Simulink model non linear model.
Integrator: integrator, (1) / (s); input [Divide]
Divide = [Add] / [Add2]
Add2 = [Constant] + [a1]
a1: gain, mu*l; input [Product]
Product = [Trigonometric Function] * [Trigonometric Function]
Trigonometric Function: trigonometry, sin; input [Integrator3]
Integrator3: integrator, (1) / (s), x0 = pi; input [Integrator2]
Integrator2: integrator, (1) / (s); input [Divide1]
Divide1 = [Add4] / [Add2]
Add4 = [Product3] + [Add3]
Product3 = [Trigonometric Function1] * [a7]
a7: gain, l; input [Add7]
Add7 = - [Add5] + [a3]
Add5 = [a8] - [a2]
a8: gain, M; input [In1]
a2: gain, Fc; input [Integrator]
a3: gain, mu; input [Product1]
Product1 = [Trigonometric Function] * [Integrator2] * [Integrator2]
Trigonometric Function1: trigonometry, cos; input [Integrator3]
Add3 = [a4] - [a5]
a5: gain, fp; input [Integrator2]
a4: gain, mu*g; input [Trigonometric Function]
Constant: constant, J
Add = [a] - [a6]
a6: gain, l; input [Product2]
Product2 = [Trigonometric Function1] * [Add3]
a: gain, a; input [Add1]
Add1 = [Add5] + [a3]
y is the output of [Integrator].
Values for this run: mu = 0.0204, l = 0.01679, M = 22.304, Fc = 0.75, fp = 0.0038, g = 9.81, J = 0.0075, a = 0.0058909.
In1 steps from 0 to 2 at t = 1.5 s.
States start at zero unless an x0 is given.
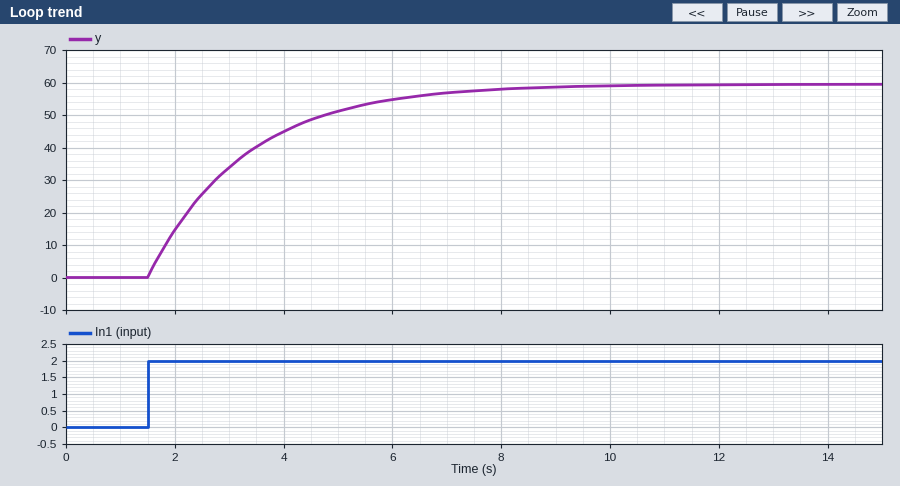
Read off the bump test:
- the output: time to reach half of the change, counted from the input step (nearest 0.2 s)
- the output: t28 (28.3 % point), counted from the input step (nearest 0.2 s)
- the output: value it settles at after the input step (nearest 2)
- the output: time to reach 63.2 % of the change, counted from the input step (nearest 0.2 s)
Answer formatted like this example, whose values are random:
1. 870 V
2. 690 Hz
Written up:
1. 1.2 s
2. 0.6 s
3. 60
4. 1.8 s
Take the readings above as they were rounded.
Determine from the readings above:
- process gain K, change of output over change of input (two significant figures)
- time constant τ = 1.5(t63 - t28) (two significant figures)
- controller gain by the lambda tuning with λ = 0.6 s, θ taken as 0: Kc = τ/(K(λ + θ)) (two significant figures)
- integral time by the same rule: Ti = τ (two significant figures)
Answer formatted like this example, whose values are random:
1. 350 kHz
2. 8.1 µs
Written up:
1. 30
2. 1.8 s
3. 0.10
4. 1.8 s
